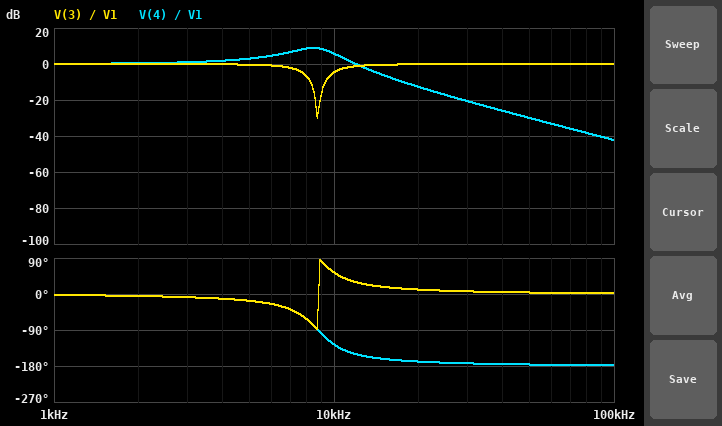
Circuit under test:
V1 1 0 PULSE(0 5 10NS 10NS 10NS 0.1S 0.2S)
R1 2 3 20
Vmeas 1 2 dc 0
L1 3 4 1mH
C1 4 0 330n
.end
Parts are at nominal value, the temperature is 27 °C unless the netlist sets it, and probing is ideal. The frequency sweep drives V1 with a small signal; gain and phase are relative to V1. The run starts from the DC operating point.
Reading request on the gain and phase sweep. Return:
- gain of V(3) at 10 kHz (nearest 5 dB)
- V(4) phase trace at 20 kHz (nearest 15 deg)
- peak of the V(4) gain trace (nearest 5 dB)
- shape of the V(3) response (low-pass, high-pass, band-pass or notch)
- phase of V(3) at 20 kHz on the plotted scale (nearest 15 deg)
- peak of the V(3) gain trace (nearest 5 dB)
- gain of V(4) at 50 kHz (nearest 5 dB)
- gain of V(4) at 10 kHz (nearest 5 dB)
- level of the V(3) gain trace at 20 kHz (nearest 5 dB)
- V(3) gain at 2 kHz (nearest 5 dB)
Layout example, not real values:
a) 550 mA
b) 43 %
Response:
a) -5 dB
b) -165 deg
c) 10 dB
d) notch
e) 15 deg
f) 0 dB
g) -30 dB
h) 5 dB
i) 0 dB
j) 0 dB
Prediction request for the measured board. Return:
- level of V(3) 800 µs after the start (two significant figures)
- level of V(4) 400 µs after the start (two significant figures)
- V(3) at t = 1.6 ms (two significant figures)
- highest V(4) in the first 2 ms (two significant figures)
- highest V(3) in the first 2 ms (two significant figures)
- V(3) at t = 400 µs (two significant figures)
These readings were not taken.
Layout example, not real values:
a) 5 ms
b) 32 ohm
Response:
a) 5.0 V
b) 5.1 V
c) 5.0 V
d) 7.8 V
e) 5.8 V
f) 5.0 V
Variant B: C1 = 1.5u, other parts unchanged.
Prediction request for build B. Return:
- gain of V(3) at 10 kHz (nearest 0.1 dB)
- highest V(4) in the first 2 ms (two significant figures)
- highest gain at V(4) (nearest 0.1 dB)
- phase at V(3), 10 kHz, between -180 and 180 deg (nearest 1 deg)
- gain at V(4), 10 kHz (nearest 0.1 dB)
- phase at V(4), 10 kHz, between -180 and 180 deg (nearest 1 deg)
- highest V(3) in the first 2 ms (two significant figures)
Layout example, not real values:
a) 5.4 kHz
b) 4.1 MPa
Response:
a) -0.6 dB
b) 6.3 V
c) 2.9 dB
d) 21 deg
e) -14.4 dB
f) -159 deg
g) 5.6 V
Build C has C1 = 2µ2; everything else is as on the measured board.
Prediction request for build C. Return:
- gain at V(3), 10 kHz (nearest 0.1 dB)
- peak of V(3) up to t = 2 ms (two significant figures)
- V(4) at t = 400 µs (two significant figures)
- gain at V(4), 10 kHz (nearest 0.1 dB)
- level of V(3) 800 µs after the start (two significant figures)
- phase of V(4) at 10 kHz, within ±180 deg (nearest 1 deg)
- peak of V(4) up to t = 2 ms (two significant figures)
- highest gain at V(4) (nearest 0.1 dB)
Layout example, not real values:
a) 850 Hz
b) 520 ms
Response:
a) -0.5 dB
b) 5.5 V
c) 4.9 V
d) -18.2 dB
e) 5.0 V
f) -160 deg
g) 5.9 V
h) 1.6 dB
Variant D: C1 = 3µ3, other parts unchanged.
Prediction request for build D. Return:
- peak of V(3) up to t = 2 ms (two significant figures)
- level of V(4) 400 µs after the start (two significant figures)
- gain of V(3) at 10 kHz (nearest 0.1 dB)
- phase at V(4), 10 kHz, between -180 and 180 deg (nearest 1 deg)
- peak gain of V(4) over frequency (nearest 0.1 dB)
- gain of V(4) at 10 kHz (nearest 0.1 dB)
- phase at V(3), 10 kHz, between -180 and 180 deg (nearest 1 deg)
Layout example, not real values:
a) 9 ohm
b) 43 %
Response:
a) 5.3 V
b) 5.0 V
c) -0.5 dB
d) -161 deg
e) 0.5 dB
f) -22.1 dB
g) 19 deg
